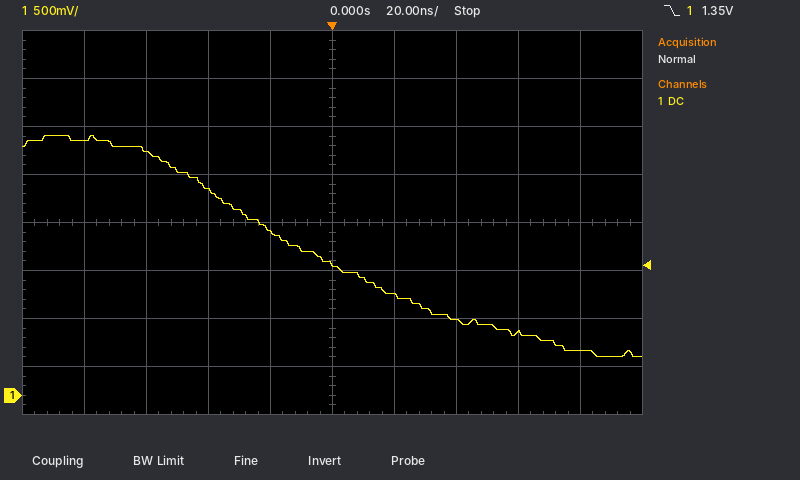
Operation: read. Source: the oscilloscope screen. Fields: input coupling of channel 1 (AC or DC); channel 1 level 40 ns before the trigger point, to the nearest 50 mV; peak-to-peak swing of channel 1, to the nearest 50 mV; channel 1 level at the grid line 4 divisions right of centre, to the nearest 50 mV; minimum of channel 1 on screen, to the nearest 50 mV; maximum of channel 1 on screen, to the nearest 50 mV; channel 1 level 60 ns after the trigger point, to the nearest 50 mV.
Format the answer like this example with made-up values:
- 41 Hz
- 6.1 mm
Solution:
- DC
- 2.15 V
- 2.30 V
- 450 mV
- 400 mV
- 2.70 V
- 650 mV
